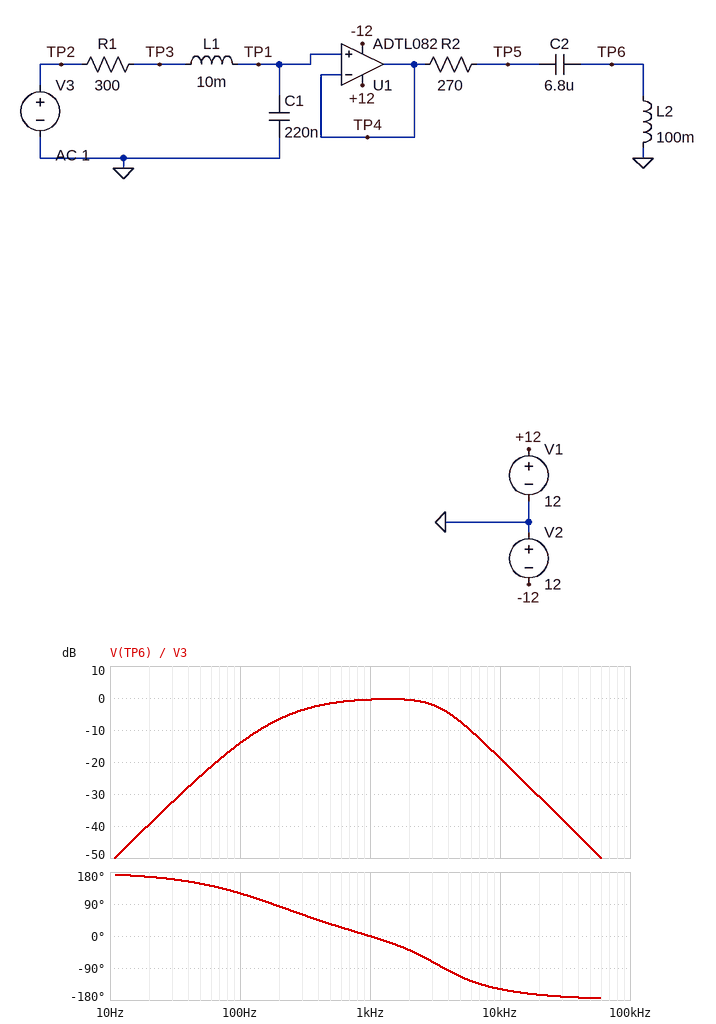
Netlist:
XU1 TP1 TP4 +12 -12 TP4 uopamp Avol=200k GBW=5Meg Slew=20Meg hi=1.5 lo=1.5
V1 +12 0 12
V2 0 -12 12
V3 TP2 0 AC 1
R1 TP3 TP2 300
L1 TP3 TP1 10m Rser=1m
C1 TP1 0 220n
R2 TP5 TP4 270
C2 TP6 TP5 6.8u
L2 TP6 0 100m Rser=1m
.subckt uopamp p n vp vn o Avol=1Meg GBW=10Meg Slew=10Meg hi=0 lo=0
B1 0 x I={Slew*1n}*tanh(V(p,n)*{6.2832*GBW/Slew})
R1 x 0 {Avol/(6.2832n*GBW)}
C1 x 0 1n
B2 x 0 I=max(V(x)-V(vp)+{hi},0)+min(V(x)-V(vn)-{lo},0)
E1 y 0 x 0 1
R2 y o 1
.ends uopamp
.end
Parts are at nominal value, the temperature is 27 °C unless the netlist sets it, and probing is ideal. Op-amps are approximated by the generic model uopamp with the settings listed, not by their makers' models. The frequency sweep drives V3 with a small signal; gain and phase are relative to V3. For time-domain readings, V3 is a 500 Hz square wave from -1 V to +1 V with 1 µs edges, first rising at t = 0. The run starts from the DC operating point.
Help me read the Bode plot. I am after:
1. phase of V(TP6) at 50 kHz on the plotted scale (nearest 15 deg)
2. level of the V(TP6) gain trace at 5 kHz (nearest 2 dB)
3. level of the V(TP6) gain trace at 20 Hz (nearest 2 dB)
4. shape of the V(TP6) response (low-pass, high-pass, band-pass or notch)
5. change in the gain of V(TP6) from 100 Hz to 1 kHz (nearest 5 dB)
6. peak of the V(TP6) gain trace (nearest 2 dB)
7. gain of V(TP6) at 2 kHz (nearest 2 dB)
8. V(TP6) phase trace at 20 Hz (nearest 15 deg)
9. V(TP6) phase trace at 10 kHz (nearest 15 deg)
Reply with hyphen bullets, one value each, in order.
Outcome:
- -180 deg
- -8 dB
- -40 dB
- band-pass
- 15 dB
- 0 dB
- 0 dB
- 165 deg
- -150 deg
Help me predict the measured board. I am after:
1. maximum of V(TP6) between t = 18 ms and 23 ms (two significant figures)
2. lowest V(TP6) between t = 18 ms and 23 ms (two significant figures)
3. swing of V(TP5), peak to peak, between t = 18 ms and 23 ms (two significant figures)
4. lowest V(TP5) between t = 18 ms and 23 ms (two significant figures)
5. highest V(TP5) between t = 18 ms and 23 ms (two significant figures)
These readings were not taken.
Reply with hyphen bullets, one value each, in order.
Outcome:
- 1.6 V
- -1.6 V
- 3.0 V
- -1.5 V
- 1.5 V
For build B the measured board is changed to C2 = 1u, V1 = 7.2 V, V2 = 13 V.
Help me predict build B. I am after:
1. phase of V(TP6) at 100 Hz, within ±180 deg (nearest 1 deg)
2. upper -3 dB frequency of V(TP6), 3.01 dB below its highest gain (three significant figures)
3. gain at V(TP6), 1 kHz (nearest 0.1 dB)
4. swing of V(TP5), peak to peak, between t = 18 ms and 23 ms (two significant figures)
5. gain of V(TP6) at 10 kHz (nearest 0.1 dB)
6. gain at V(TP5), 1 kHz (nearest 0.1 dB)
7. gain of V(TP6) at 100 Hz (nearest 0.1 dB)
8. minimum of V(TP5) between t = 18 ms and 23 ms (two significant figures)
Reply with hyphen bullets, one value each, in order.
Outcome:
- 168 deg
- 2.44 kHz
- 1.3 dB
- 1.4 V
- -18.8 dB
- -1.3 dB
- -27.9 dB
- -690 mV
